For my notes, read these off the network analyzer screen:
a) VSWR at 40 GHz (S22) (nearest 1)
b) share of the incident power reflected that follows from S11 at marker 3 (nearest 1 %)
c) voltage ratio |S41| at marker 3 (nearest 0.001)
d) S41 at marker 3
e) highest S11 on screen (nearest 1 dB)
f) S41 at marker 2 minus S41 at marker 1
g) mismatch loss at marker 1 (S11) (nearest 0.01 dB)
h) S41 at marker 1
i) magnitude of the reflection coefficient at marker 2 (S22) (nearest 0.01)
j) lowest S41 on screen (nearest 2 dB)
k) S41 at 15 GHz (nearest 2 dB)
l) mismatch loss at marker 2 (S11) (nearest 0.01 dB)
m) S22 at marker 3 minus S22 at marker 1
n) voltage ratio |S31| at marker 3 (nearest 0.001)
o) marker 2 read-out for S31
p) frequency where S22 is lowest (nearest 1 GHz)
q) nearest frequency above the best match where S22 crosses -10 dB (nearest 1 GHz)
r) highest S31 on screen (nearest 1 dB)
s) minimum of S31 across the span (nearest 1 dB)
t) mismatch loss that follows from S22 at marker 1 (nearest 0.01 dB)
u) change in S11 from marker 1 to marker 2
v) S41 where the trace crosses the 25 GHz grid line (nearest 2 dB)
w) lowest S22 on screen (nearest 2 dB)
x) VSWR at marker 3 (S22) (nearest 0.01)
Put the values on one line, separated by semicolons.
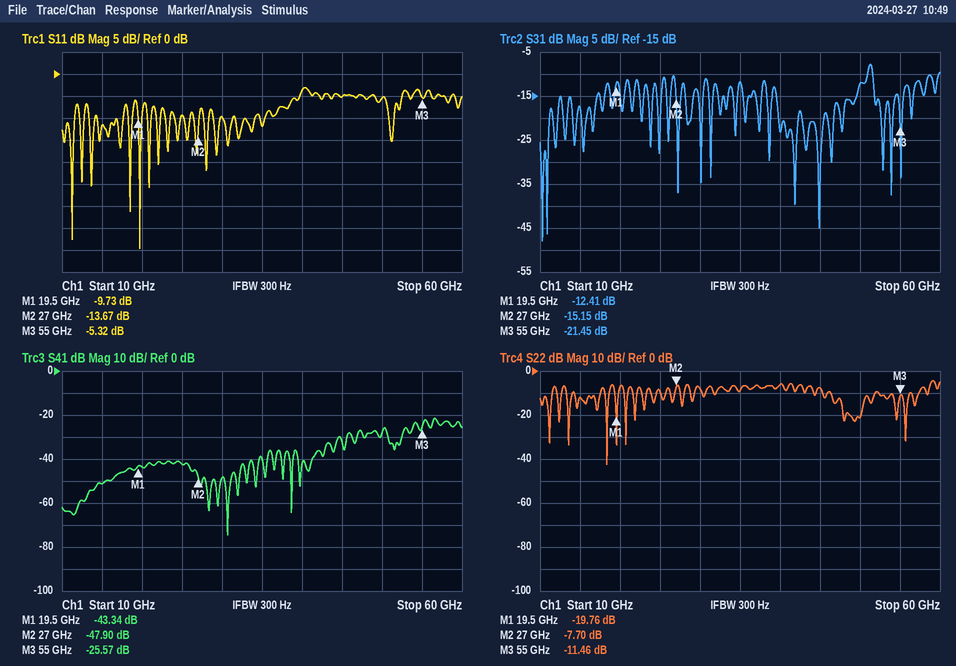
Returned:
3; 29 %; 0.053; -25.57 dB; -3 dB; -4.56 dB; 0.49 dB; -43.34 dB; 0.41; -74 dB; -52 dB; 0.19 dB; 8.30 dB; 0.085; -15.15 dB; 18 GHz; 19 GHz; -8 dB; -48 dB; 0.05 dB; -3.94 dB; -42 dB; -42 dB; 1.73
